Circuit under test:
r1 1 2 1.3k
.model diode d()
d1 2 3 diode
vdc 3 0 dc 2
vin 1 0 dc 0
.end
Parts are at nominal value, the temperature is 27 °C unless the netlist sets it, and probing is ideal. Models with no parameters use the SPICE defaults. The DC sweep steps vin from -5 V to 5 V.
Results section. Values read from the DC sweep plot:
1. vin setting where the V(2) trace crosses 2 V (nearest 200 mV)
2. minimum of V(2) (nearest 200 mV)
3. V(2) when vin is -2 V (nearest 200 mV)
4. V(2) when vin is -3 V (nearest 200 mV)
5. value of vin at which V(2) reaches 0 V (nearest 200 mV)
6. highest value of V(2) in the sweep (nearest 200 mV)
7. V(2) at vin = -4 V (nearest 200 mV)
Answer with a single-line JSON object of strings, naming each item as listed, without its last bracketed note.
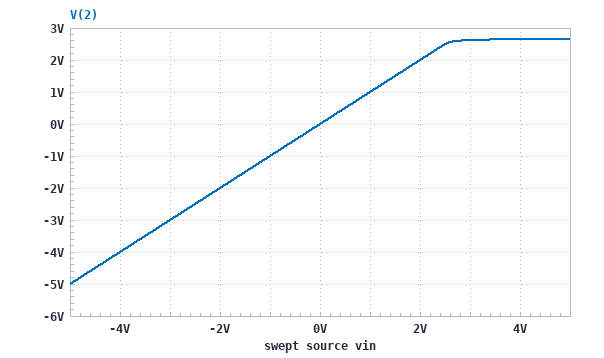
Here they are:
{"vin setting where the V(2) trace crosses 2 V": "2.0 V", "minimum of V(2)": "-5.0 V", "V(2) when vin is -2 V": "-2.0 V", "V(2) when vin is -3 V": "-3.0 V", "value of vin at which V(2) reaches 0 V": "0 V", "highest value of V(2) in the sweep": "2.6 V", "V(2) at vin = -4 V": "-4.0 V"}
